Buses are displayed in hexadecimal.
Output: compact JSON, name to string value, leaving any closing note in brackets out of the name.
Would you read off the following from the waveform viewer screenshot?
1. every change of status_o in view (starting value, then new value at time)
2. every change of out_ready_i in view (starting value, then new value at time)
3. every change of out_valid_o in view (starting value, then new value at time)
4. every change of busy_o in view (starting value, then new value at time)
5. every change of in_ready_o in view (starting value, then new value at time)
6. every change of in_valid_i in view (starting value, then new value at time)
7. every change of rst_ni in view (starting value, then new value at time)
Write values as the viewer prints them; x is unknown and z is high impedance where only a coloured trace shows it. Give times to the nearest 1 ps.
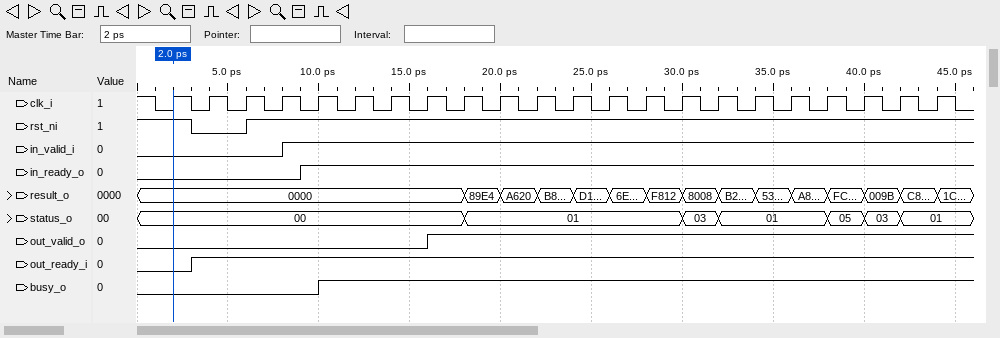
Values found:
{"every change of status_o in view": "00, 01 at 18 ps, 03 at 30 ps, 01 at 32 ps, 05 at 38 ps, 03 at 40 ps, 01 at 42 ps", "every change of out_ready_i in view": "0, 1 at 3 ps", "every change of out_valid_o in view": "0, 1 at 16 ps", "every change of busy_o in view": "0, 1 at 10 ps", "every change of in_ready_o in view": "0, 1 at 9 ps", "every change of in_valid_i in view": "0, 1 at 8 ps", "every change of rst_ni in view": "1, 0 at 3 ps, 1 at 6 ps"}
